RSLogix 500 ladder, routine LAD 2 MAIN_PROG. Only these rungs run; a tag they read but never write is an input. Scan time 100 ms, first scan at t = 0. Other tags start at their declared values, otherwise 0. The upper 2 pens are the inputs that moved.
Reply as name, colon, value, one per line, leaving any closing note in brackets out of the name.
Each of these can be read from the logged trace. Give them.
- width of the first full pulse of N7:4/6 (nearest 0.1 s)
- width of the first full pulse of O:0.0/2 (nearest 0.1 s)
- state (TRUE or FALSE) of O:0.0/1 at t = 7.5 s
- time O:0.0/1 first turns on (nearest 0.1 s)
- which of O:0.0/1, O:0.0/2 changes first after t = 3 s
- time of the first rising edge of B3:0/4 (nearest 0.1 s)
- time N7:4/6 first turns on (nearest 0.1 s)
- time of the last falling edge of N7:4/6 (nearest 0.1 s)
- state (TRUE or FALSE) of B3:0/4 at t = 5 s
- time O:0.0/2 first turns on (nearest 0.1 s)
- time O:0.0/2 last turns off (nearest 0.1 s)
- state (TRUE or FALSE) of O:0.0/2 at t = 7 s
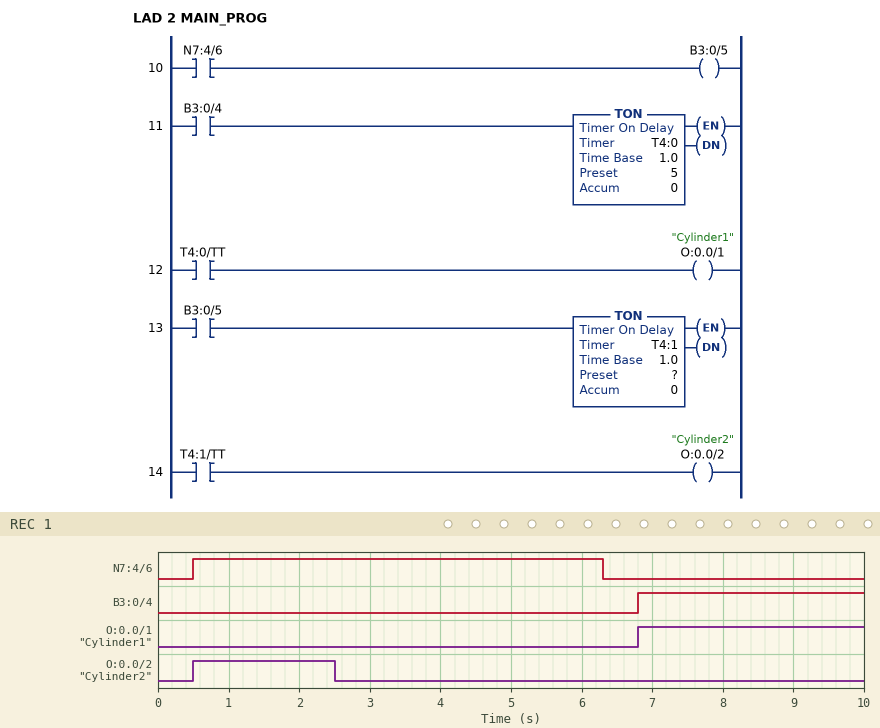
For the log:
width of the first full pulse of N7:4/6: 5.8 s
width of the first full pulse of O:0.0/2: 2.0 s
state (TRUE or FALSE) of O:0.0/1 at t = 7.5 s: TRUE
time O:0.0/1 first turns on: 6.8 s
which of O:0.0/1, O:0.0/2 changes first after t = 3 s: O:0.0/1
time of the first rising edge of B3:0/4: 6.8 s
time N7:4/6 first turns on: 0.5 s
time of the last falling edge of N7:4/6: 6.3 s
state (TRUE or FALSE) of B3:0/4 at t = 5 s: FALSE
time O:0.0/2 first turns on: 0.5 s
time O:0.0/2 last turns off: 2.5 s
state (TRUE or FALSE) of O:0.0/2 at t = 7 s: FALSE
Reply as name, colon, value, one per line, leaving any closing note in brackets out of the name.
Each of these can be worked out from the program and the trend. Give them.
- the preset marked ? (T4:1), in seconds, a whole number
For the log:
the preset marked ? (T4:1), in seconds, a whole number: 2 s
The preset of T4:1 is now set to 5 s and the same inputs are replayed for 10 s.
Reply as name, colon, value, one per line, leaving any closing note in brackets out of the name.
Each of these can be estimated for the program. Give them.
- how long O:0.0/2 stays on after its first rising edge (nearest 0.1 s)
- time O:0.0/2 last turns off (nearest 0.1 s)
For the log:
how long O:0.0/2 stays on after its first rising edge: 5.0 s
time O:0.0/2 last turns off: 5.5 s
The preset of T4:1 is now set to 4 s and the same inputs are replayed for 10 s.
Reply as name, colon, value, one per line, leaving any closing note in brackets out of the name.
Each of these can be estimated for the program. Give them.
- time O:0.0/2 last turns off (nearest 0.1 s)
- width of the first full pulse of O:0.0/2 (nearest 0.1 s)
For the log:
time O:0.0/2 last turns off: 4.5 s
width of the first full pulse of O:0.0/2: 4.0 s
